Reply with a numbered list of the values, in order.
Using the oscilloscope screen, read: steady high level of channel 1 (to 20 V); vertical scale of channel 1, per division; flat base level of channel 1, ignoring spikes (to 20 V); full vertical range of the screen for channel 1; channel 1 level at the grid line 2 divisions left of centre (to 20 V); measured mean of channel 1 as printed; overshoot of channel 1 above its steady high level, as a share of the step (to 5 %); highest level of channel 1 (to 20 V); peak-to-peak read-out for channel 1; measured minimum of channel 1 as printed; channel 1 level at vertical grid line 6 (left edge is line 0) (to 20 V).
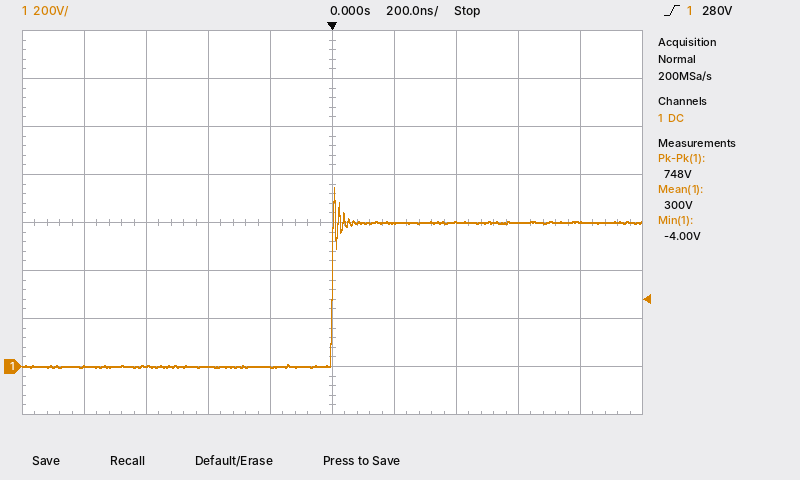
1. 600 V
2. 200 V
3. 0 V
4. 1.6 kV
5. 0 V
6. 300 V
7. 25 %
8. 740 V
9. 748 V
10. -4.00 V
11. 600 V
